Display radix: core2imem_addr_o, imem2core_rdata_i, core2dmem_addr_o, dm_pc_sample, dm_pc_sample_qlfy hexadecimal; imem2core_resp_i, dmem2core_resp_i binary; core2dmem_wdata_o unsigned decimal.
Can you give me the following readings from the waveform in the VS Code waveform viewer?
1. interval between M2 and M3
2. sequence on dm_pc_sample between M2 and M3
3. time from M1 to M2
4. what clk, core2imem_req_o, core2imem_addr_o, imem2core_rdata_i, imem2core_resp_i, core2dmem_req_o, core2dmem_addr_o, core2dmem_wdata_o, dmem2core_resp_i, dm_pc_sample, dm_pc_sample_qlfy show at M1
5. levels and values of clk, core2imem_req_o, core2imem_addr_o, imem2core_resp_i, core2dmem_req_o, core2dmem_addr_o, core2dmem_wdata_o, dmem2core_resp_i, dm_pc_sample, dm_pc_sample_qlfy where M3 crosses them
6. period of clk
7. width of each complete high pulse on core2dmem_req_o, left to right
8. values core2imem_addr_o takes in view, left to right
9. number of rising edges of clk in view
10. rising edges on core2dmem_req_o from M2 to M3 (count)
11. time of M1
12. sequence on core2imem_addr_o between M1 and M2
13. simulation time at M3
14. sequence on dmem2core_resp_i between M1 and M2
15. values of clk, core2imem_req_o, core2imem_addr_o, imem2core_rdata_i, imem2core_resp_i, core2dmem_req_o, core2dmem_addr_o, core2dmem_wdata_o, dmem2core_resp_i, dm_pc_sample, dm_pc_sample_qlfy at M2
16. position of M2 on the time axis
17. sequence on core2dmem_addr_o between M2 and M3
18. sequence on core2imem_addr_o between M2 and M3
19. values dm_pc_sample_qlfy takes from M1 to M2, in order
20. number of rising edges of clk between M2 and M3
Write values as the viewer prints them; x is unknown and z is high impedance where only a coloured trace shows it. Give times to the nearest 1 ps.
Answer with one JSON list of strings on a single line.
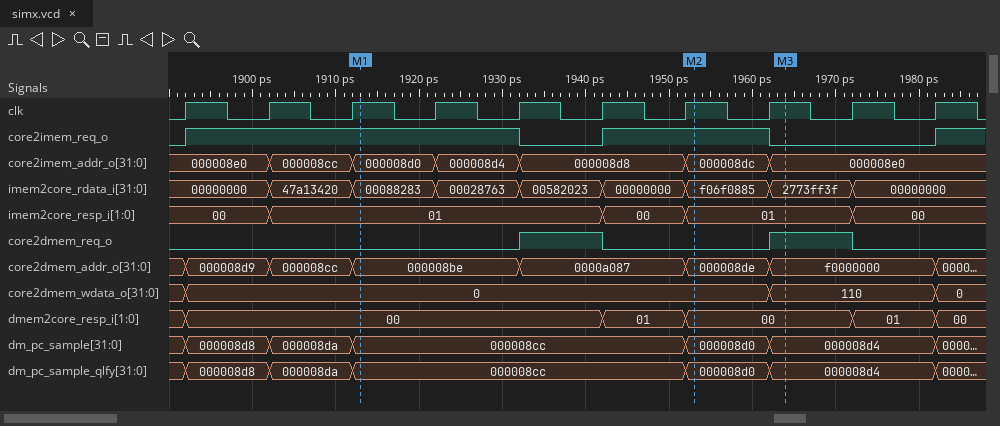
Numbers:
["11 ps", "000008d0, 000008d4", "40 ps", "clk=1, core2imem_req_o=1, core2imem_addr_o=000008d0, imem2core_rdata_i=00088283, imem2core_resp_i=01, core2dmem_req_o=0, core2dmem_addr_o=000008be, core2dmem_wdata_o=0, dmem2core_resp_i=00, dm_pc_sample=000008cc, dm_pc_sample_qlfy=000008cc", "clk=1, core2imem_req_o=0, core2imem_addr_o=000008e0, imem2core_resp_i=01, core2dmem_req_o=1, core2dmem_addr_o=f0000000, core2dmem_wdata_o=110, dmem2core_resp_i=00, dm_pc_sample=000008d4, dm_pc_sample_qlfy=000008d4", "10 ps", "10 ps, 10 ps", "000008e0, 000008cc, 000008d0, 000008d4, 000008d8, 000008dc, 000008e0", "10", "1", "1913 ps", "000008d0, 000008d4, 000008d8, 000008dc", "1964 ps", "00, 01, 00", "clk=1, core2imem_req_o=1, core2imem_addr_o=000008dc, imem2core_rdata_i=f06f0885, imem2core_resp_i=01, core2dmem_req_o=0, core2dmem_addr_o=000008de, core2dmem_wdata_o=0, dmem2core_resp_i=00, dm_pc_sample=000008d0, dm_pc_sample_qlfy=000008d0", "1953 ps", "000008de, f0000000", "000008dc, 000008e0", "000008cc, 000008d0", "1"]
